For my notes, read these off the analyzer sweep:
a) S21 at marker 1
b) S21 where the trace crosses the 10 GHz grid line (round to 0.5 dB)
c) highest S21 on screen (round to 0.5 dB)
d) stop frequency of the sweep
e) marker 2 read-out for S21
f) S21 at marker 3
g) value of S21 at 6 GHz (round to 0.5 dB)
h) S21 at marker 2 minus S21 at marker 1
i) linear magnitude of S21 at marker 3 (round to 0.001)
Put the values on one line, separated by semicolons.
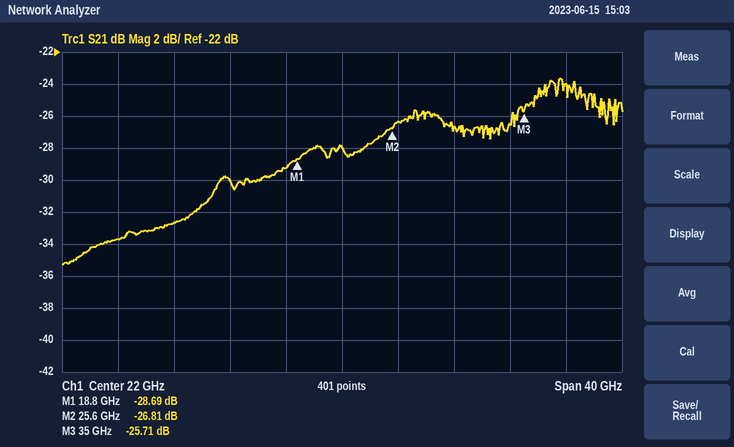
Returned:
-28.69 dB; -32.5 dB; -23.5 dB; 42 GHz; -26.81 dB; -25.71 dB; -33.5 dB; 1.88 dB; 0.052
